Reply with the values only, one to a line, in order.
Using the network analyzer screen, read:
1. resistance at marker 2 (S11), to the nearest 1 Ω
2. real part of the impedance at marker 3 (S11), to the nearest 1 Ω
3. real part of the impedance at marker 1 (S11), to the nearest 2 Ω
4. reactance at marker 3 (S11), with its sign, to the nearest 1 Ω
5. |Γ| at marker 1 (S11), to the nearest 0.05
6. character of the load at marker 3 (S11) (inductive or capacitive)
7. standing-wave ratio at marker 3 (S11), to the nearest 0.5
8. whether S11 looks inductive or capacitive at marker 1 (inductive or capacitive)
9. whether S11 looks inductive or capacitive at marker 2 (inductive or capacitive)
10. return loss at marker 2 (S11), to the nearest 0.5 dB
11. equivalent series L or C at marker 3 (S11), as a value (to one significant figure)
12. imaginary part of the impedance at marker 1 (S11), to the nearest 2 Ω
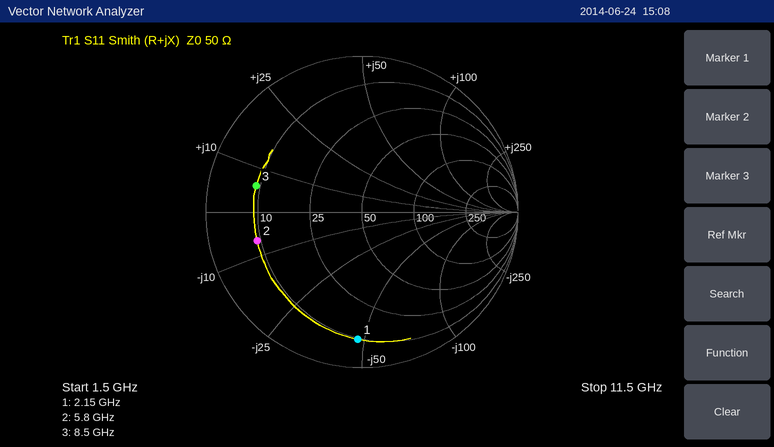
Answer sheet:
9 Ω
9 Ω
10 Ω
+6 Ω
0.80
inductive
5.5
capacitive
capacitive
3.0 dB
100 pH
-48 Ω
